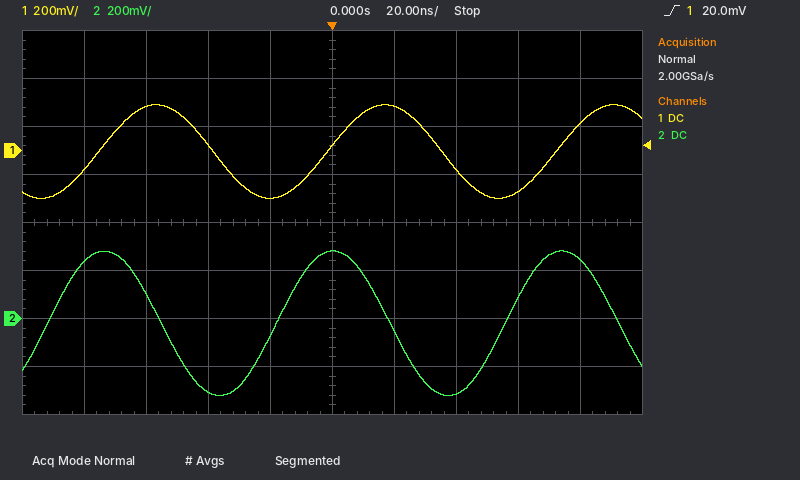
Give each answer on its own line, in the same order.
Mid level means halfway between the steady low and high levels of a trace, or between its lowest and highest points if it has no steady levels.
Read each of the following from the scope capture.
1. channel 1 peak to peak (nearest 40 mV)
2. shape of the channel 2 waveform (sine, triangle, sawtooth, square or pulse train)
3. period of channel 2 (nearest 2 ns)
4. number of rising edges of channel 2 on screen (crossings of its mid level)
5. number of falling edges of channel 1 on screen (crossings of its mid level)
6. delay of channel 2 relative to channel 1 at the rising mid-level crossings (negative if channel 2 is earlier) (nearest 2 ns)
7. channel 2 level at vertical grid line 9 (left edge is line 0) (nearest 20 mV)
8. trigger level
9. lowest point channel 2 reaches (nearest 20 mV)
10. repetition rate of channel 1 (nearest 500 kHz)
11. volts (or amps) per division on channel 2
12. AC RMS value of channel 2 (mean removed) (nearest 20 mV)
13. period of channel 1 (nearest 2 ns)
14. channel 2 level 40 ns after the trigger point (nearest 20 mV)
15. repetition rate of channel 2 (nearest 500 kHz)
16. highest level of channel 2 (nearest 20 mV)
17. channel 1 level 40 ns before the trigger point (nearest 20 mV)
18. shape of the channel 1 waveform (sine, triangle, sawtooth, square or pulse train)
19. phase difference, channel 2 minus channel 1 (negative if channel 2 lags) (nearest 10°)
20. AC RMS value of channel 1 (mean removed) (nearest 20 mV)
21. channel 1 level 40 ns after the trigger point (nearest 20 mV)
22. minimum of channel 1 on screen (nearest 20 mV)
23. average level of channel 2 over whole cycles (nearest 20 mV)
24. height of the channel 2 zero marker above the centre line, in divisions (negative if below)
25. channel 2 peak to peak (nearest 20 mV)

400 mV
sine
74 ns
3
2
-16 ns
240 mV
20.0 mV
-320 mV
13.5 MHz
200 mV
220 mV
74 ns
-320 mV
13.5 MHz
280 mV
20 mV
sine
+80°
140 mV
-80 mV
-200 mV
-20 mV
-2.0 div
600 mV
